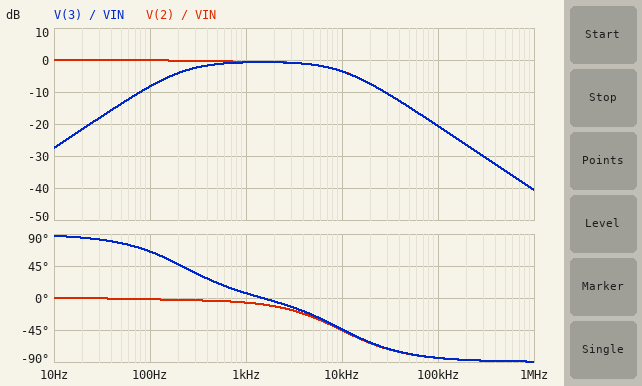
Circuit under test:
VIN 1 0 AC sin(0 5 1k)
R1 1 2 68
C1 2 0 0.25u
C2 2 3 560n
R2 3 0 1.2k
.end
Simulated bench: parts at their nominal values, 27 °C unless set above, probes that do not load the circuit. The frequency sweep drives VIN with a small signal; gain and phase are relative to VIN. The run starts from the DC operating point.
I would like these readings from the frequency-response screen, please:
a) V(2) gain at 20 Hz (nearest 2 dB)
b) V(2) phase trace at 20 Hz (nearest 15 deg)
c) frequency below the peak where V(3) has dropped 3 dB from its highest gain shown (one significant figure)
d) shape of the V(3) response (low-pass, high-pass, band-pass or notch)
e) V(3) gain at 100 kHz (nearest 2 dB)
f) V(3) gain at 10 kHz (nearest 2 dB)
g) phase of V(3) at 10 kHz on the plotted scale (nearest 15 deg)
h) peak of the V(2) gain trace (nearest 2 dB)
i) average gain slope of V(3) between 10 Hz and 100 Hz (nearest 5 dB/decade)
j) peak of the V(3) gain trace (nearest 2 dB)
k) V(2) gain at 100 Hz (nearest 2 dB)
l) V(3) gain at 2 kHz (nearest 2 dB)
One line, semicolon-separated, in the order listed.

0 dB; 0 deg; 200 Hz; band-pass; -20 dB; -4 dB; -45 deg; 0 dB; 20 dB/decade; 0 dB; 0 dB; 0 dB
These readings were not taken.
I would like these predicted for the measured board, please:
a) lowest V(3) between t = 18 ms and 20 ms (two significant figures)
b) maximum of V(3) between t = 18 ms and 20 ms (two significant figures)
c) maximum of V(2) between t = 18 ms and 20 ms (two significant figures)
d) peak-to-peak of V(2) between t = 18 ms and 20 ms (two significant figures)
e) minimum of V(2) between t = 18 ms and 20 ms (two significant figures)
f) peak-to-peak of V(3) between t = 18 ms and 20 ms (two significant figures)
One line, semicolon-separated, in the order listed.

-4.6 V; 4.6 V; 4.7 V; 9.4 V; -4.7 V; 9.2 V
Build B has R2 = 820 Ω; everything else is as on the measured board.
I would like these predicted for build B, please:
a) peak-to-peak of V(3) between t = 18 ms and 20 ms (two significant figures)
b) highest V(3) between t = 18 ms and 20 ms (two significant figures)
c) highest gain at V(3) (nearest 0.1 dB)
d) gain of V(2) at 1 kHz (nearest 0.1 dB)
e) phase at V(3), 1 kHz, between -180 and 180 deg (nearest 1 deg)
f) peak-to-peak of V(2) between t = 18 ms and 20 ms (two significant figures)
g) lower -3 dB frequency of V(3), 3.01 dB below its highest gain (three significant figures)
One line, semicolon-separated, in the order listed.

8.7 V; 4.4 V; -1.0 dB; -0.7 dB; 12 deg; 9.2 V; 301 Hz
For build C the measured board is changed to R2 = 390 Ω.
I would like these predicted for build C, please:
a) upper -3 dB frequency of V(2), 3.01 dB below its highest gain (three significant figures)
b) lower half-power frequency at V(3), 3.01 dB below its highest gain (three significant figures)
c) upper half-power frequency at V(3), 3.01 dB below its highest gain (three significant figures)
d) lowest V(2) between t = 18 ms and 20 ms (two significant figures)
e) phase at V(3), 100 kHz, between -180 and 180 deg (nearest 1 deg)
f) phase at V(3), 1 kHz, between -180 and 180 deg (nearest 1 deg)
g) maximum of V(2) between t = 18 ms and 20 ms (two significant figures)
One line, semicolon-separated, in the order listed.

7.24 kHz; 556 Hz; 12.3 kHz; -4.4 V; -83 deg; 26 deg; 4.4 V
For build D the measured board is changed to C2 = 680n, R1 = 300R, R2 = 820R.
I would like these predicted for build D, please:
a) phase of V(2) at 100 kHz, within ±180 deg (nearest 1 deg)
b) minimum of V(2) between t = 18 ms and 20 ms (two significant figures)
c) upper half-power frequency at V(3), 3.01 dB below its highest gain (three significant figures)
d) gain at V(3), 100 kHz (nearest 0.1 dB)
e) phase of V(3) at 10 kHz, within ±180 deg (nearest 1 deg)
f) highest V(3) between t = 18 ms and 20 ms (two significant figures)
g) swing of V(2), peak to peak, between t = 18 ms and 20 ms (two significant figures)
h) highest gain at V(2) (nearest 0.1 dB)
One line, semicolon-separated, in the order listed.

-88 deg; -3.4 V; 3.36 kHz; -33.5 dB; -72 deg; 3.3 V; 6.9 V; 0 dB
